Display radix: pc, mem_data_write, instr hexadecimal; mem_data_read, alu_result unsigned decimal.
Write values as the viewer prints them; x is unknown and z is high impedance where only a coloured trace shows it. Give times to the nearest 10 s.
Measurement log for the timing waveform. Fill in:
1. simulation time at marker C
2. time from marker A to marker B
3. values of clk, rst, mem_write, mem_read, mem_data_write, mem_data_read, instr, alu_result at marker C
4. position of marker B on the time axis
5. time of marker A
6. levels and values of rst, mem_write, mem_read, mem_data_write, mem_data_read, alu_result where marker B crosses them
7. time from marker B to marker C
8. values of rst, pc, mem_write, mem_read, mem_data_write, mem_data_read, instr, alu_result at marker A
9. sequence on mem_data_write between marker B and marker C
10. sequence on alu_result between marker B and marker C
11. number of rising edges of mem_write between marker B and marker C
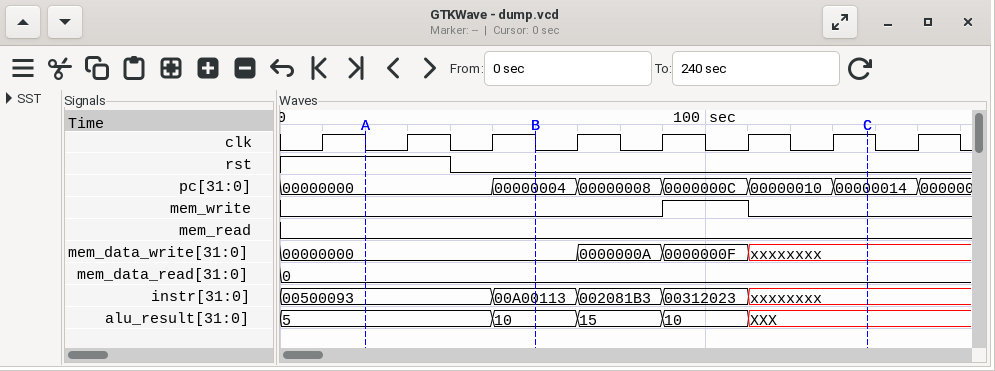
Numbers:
140 s
40 s
clk=1, rst=0, mem_write=0, mem_read=0, mem_data_write=xxxxxxxx, mem_data_read=0, instr=xxxxxxxx, alu_result=XXX
60 s
20 s
rst=0, mem_write=0, mem_read=0, mem_data_write=00000000, mem_data_read=0, alu_result=10
80 s
rst=1, pc=00000000, mem_write=0, mem_read=0, mem_data_write=00000000, mem_data_read=0, instr=00500093, alu_result=5
00000000, 0000000A, 0000000F, xxxxxxxx
10, 15, 10, XXX
1
